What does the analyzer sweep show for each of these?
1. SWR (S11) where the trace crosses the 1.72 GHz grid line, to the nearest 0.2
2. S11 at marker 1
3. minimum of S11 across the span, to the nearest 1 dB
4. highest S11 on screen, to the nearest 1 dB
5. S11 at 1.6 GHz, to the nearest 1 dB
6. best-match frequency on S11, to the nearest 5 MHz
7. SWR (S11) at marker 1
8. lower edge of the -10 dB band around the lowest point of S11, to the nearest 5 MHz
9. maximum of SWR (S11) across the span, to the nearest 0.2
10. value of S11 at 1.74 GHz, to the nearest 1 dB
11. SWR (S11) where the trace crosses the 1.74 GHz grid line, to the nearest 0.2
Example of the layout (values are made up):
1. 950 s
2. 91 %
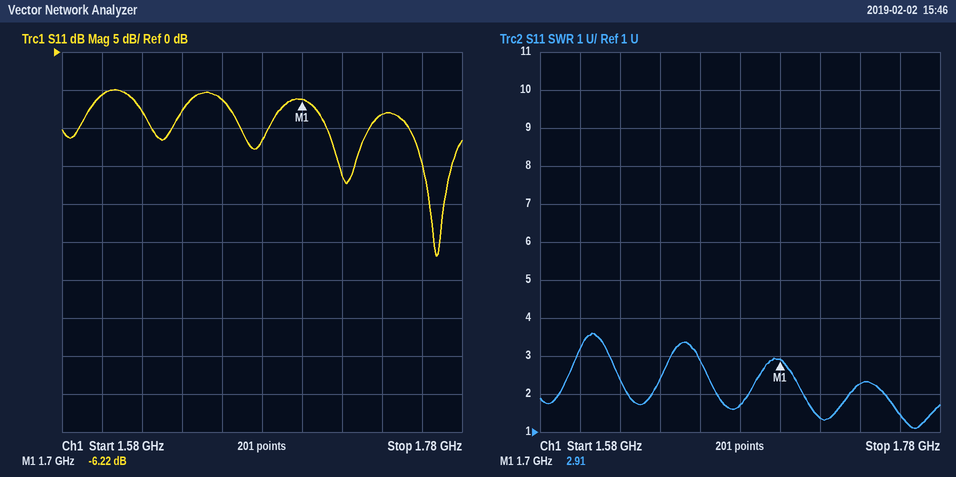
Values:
1. 1.4
2. -6.22 dB
3. -27 dB
4. -5 dB
5. -6 dB
6. 1.765 GHz
7. 2.91
8. 1.755 GHz
9. 3.6
10. -8 dB
11. 2.2
